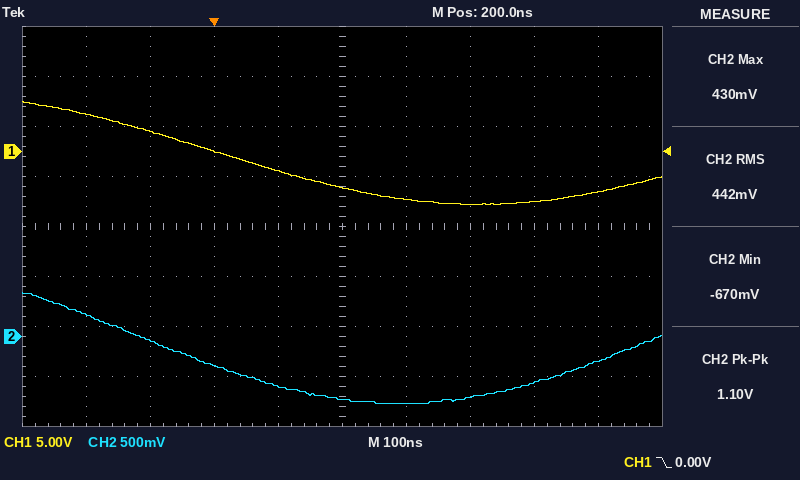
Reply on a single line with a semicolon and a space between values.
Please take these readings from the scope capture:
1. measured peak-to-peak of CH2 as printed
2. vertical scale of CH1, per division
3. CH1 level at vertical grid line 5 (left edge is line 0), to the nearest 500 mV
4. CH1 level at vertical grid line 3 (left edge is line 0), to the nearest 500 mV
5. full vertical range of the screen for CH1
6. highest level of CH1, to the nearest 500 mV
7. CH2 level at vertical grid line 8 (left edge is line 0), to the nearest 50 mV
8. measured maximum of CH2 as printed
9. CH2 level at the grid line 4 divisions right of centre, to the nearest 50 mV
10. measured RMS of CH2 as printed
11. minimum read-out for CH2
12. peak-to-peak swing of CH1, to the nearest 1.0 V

1.10 V; 5 V; -3.5 V; 0.0 V; 40 V; 5.0 V; -450 mV; 430 mV; -250 mV; 442 mV; -670 mV; 10.0 V
